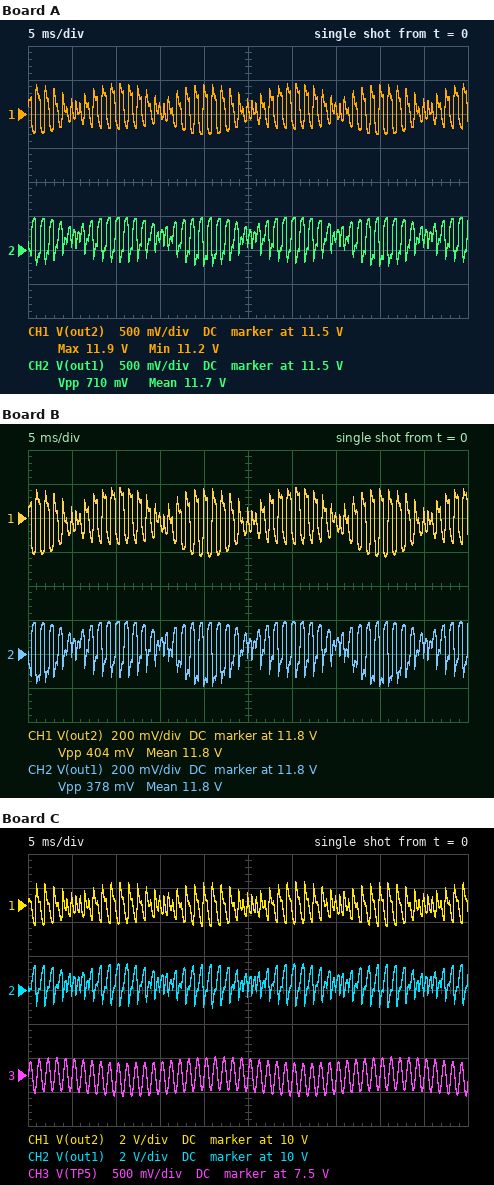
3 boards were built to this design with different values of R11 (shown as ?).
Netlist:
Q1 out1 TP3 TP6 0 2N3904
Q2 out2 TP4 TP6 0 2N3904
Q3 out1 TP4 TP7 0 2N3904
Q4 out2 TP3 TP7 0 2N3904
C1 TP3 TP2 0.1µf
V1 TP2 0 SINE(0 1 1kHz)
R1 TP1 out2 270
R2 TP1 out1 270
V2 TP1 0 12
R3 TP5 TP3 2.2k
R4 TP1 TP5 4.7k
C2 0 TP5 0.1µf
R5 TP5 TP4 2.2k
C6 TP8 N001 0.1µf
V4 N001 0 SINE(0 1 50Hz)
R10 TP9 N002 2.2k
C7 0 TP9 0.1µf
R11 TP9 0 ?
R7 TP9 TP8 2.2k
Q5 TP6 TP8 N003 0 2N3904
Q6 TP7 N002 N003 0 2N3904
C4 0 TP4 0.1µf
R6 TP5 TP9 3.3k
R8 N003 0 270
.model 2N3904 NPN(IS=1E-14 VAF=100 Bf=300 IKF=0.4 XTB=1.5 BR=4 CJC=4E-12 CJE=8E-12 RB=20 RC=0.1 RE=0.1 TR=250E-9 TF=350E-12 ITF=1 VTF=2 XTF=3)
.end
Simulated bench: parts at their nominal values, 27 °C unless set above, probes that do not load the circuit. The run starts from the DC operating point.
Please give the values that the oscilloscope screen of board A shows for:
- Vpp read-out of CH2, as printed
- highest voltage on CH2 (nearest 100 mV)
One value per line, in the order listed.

710 mV
12.0 V
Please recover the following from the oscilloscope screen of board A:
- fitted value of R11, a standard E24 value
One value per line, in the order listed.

1.1 kΩ
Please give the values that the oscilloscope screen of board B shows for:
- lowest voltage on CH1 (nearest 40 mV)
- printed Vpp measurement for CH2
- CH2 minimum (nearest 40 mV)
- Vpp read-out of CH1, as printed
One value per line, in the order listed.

11.56 V
378 mV
11.60 V
404 mV
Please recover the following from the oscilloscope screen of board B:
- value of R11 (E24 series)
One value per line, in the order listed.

750 Ω
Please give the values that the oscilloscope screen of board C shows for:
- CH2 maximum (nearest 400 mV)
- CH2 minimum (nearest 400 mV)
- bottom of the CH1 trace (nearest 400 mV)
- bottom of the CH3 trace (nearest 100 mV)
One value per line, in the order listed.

11.6 V
8.8 V
8.8 V
7.2 V
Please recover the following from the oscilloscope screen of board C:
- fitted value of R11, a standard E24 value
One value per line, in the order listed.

5.1 kΩ
